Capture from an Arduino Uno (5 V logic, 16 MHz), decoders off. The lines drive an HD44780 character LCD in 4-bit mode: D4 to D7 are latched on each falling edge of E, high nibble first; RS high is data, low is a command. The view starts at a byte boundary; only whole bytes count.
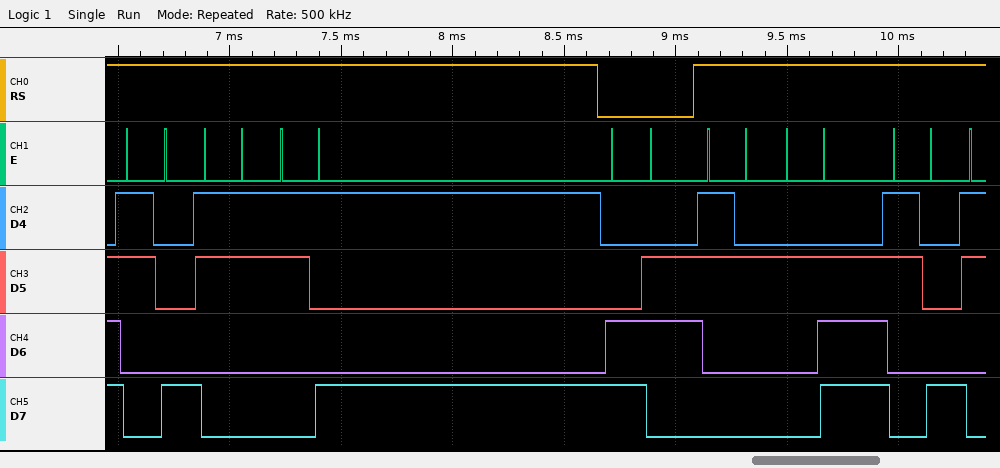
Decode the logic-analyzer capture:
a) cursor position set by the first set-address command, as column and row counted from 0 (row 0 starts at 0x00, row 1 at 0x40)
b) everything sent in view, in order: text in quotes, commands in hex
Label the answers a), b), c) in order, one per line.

a) column 6, row 1
b) "839" 0xC6 "2.8"
